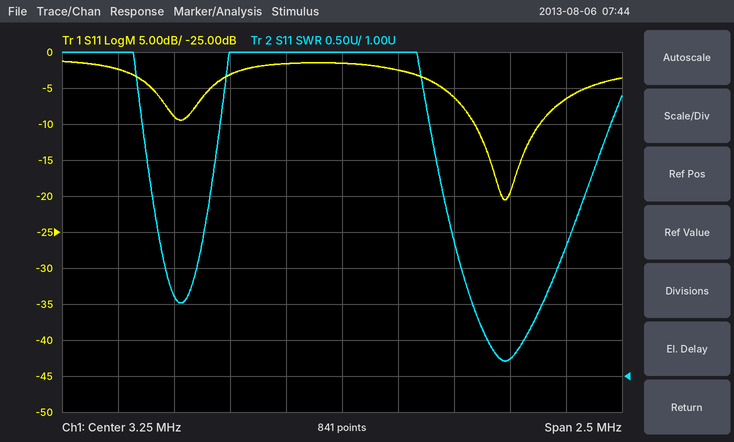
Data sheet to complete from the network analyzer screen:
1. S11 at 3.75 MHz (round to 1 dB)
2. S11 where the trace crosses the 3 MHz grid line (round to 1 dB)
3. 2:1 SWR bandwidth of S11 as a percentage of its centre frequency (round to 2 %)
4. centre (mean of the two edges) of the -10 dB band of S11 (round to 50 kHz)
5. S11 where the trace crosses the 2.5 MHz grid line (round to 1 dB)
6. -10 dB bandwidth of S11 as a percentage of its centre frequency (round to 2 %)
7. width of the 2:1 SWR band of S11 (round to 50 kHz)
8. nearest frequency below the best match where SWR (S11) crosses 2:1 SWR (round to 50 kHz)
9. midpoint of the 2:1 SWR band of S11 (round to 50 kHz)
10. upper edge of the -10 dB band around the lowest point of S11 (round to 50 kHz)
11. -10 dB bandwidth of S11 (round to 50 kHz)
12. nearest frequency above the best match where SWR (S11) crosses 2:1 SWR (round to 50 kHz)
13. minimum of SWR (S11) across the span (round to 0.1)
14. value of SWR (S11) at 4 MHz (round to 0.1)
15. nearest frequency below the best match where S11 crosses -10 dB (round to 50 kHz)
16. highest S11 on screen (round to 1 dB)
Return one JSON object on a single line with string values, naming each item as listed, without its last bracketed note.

{"S11 at 3.75 MHz": "-6 dB", "S11 where the trace crosses the 3 MHz grid line": "-2 dB", "2:1 SWR bandwidth of S11 as a percentage of its centre frequency": "8 %", "centre (mean of the two edges) of the -10 dB band of S11": "4.00 MHz", "S11 where the trace crosses the 2.5 MHz grid line": "-9 dB", "-10 dB bandwidth of S11 as a percentage of its centre frequency": "8 %", "width of the 2:1 SWR band of S11": "300 kHz", "nearest frequency below the best match where SWR (S11) crosses 2:1 SWR": "3.85 MHz", "midpoint of the 2:1 SWR band of S11": "4.00 MHz", "upper edge of the -10 dB band around the lowest point of S11": "4.15 MHz", "-10 dB bandwidth of S11": "300 kHz", "nearest frequency above the best match where SWR (S11) crosses 2:1 SWR": "4.15 MHz", "minimum of SWR (S11) across the span": "1.2", "value of SWR (S11) at 4 MHz": "1.2", "nearest frequency below the best match where S11 crosses -10 dB": "3.85 MHz", "highest S11 on screen": "-1 dB"}
